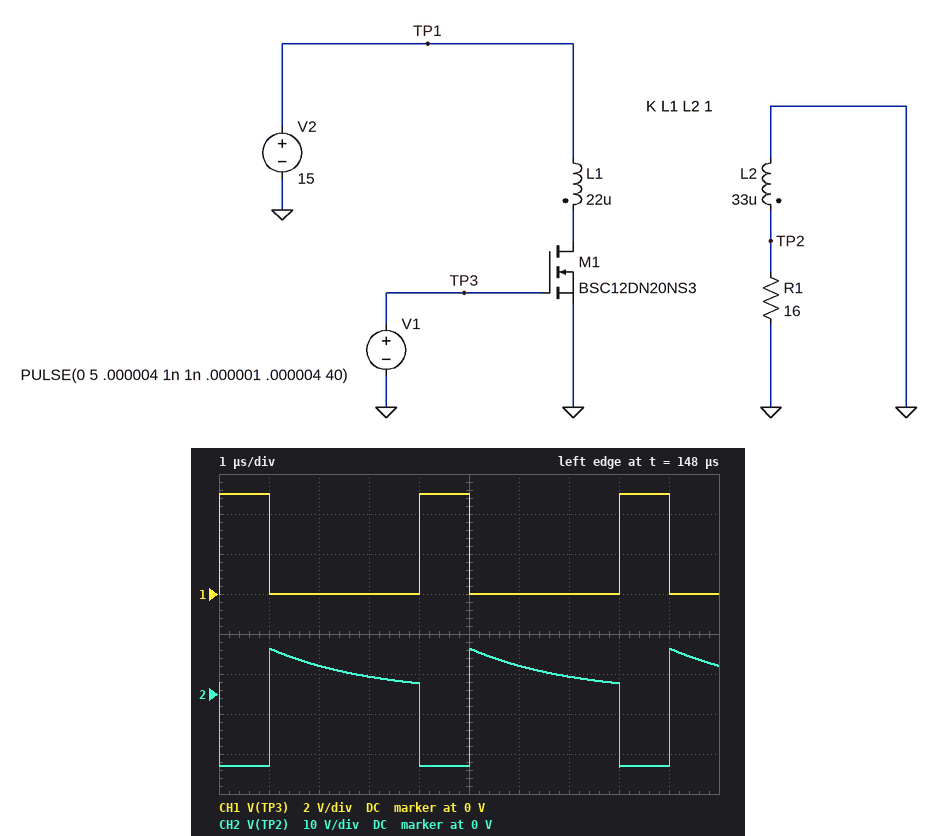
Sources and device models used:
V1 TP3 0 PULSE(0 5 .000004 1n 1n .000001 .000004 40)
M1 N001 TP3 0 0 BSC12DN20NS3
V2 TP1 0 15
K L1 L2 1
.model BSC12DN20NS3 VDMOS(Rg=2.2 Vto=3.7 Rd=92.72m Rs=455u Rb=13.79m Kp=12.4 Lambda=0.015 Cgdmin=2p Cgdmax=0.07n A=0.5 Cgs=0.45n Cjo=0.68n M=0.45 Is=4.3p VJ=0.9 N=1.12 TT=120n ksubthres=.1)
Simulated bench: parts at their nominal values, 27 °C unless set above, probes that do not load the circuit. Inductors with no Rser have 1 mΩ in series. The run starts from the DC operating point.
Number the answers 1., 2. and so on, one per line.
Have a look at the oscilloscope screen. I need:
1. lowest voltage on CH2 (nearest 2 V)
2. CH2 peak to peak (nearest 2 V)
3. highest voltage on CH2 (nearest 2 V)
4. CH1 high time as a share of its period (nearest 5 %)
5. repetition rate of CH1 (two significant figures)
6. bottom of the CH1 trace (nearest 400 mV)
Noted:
1. -18 V
2. 30 V
3. 12 V
4. 25 %
5. 250 kHz
6. 0 V
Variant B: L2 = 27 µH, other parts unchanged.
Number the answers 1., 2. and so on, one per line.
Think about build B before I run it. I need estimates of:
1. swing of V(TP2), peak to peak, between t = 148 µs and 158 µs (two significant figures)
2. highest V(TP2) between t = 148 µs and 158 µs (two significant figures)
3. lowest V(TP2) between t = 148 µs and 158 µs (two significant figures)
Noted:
1. 28 V
2. 12 V
3. -16 V
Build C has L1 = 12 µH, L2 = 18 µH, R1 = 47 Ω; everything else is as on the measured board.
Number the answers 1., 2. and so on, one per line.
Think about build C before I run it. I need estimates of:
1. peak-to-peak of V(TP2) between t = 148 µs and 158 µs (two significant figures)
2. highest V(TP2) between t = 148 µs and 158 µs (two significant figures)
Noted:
1. 64 V
2. 46 V
